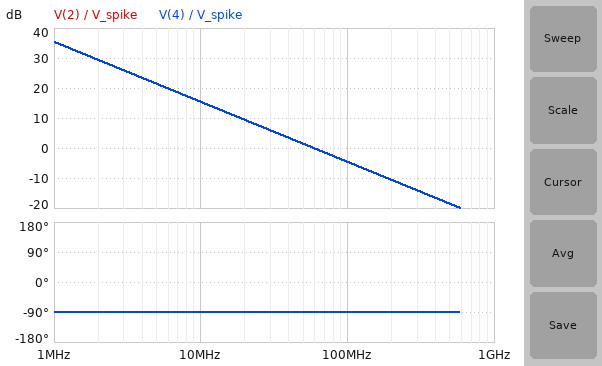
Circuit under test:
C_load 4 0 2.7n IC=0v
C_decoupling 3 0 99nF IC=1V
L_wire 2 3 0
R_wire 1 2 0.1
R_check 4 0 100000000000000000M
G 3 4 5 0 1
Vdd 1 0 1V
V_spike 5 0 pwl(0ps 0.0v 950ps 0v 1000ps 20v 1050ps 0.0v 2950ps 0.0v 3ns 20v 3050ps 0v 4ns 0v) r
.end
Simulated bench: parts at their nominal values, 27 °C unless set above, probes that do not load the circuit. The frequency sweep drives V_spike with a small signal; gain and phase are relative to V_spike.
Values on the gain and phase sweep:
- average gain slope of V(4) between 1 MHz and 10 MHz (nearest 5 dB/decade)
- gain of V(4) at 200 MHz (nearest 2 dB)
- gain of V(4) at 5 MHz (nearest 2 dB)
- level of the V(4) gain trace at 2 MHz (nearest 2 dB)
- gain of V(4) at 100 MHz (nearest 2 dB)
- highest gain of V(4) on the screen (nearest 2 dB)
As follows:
-20 dB/decade
-10 dB
22 dB
30 dB
-4 dB
36 dB
